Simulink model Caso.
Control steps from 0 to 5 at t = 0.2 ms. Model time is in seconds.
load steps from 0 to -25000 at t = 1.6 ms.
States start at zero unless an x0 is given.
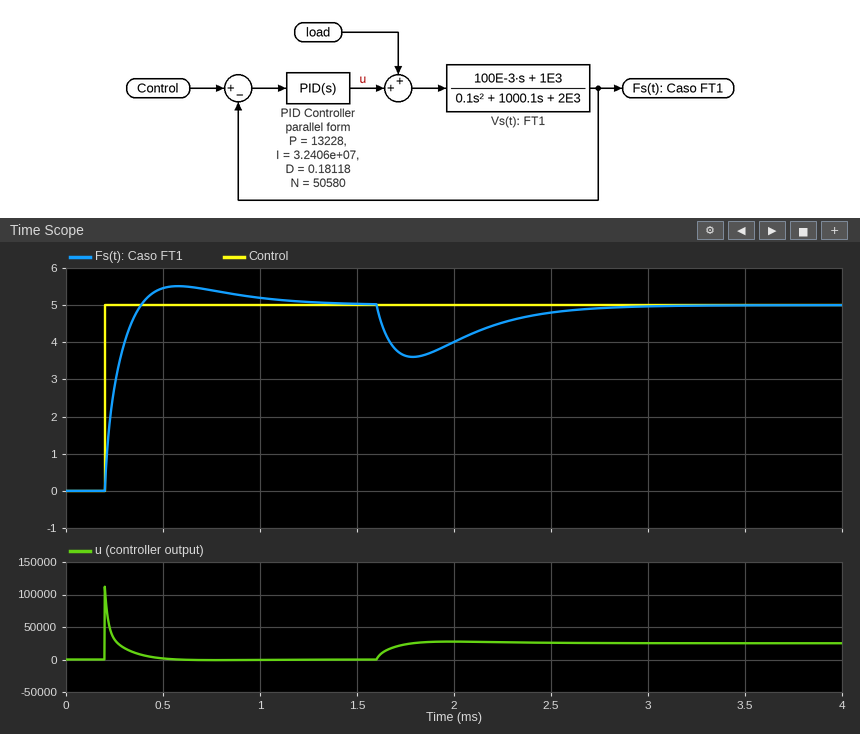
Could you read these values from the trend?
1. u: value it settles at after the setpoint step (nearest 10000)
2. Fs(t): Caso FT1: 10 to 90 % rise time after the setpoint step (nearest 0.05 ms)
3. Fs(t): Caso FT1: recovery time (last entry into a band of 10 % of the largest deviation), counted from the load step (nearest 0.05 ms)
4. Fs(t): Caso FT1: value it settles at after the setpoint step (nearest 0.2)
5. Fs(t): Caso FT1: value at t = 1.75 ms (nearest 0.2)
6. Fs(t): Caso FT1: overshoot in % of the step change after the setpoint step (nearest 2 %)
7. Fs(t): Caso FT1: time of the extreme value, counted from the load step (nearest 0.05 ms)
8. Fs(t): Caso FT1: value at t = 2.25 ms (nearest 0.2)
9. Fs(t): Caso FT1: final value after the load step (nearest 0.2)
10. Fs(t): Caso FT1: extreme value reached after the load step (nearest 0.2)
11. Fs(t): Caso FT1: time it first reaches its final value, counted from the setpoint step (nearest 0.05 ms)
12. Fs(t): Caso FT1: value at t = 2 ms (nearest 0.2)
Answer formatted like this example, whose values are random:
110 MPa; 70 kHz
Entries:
0; 0.15 ms; 1.00 ms; 5.0; 3.6; 10 %; 0.20 ms; 4.6; 5.0; 3.6; 0.20 ms; 4.0
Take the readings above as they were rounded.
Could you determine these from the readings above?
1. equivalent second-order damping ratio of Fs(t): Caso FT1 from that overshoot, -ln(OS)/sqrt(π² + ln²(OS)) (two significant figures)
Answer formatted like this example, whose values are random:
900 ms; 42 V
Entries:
0.59
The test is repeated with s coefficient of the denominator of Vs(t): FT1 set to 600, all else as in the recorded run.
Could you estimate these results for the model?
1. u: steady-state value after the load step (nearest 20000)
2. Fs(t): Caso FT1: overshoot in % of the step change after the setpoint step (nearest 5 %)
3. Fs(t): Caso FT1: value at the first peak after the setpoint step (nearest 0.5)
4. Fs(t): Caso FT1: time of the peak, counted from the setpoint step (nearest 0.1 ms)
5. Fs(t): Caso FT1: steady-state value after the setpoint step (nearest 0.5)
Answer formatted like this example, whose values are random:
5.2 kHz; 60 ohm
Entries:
20000; 15 %; 5.5; 0.3 ms; 5.0
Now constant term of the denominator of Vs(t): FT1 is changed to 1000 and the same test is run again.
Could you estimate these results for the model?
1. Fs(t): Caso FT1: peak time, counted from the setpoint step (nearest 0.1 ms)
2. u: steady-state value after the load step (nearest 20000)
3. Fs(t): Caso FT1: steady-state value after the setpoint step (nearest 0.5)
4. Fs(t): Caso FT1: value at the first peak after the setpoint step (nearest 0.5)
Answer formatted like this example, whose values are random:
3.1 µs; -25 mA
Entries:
0.4 ms; 20000; 5.0; 5.5
